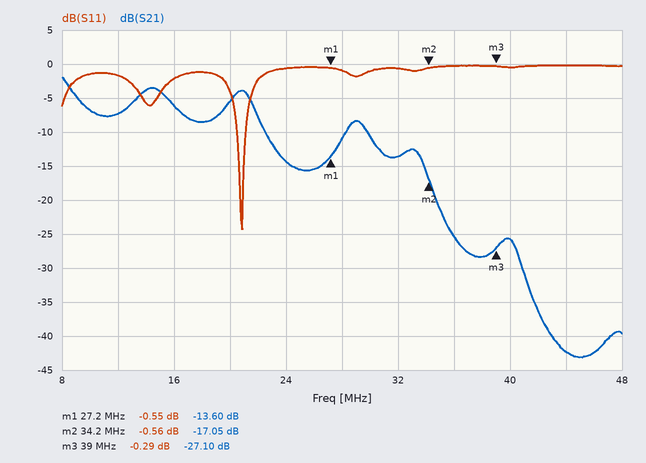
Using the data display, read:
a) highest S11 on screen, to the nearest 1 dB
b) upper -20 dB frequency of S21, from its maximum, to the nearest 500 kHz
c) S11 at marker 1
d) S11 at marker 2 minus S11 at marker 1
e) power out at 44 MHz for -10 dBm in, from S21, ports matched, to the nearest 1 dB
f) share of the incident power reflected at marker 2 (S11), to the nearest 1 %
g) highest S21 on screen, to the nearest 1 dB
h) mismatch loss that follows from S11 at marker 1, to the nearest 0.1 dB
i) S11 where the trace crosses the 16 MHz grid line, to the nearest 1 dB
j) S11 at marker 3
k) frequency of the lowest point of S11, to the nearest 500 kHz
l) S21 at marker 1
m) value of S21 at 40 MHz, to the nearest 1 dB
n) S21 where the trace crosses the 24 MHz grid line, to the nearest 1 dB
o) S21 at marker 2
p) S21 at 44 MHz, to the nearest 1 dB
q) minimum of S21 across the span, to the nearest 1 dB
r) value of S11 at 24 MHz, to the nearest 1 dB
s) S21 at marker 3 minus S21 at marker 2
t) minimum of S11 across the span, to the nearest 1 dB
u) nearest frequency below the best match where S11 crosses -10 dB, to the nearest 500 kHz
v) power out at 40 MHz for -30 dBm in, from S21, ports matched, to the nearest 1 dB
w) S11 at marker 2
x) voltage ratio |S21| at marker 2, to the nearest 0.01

0 dB
35.0 MHz
-0.55 dB
-0.01 dB
-52 dBm
88 %
-2 dB
9.2 dB
-2 dB
-0.29 dB
21.0 MHz
-13.60 dB
-26 dB
-14 dB
-17.05 dB
-42 dB
-43 dB
-1 dB
-10.05 dB
-24 dB
20.5 MHz
-56 dBm
-0.56 dB
0.14
